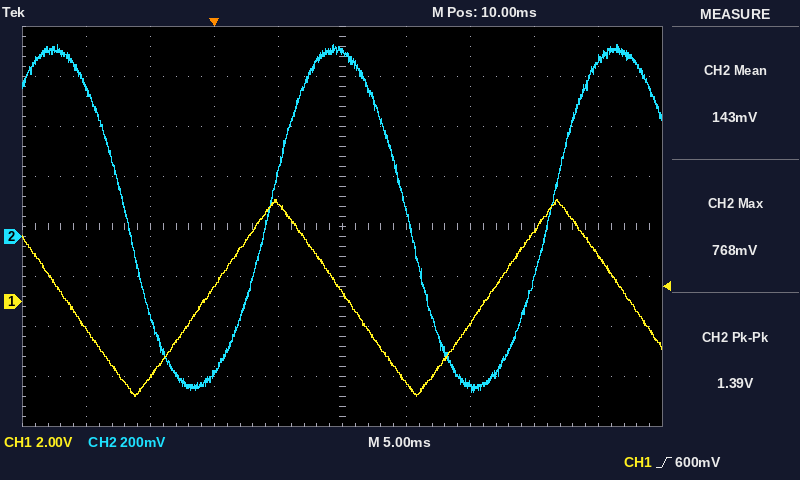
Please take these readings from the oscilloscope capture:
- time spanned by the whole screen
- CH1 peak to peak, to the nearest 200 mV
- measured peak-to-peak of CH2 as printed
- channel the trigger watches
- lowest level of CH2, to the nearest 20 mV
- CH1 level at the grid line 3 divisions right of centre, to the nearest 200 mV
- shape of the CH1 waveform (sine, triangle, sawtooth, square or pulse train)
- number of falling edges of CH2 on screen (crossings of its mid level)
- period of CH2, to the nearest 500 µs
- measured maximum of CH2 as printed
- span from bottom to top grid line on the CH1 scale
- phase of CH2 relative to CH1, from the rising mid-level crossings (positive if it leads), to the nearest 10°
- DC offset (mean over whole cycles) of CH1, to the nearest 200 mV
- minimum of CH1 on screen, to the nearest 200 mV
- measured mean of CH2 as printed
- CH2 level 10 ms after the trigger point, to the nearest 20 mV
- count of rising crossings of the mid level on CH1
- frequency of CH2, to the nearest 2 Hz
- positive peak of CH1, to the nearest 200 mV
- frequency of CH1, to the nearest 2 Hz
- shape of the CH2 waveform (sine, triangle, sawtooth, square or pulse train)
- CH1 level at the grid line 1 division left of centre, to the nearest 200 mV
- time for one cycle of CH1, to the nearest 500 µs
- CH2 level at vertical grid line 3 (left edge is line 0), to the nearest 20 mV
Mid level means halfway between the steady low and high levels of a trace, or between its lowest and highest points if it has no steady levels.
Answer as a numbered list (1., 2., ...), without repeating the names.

1. 50 ms
2. 7.8 V
3. 1.39 V
4. CH1
5. -620 mV
6. 2.8 V
7. triangle
8. 2
9. 22.0 ms
10. 768 mV
11. 16 V
12. -80°
13. 200 mV
14. -3.8 V
15. 143 mV
16. 740 mV
17. 2
18. 46 Hz
19. 4.0 V
20. 46 Hz
21. sine
22. 4.0 V
23. 22.0 ms
24. -540 mV
